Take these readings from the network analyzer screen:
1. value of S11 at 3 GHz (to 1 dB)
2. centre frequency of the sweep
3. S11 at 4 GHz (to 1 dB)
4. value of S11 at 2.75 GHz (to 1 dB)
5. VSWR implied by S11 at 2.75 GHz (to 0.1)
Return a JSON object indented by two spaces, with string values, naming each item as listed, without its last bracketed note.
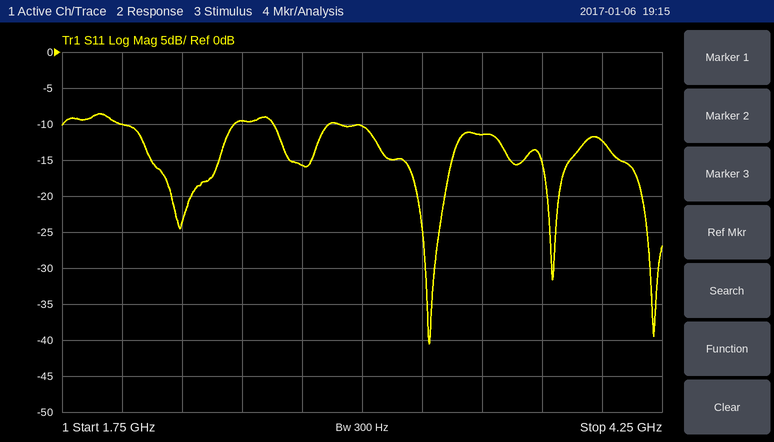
{
  "value of S11 at 3 GHz": "-10 dB",
  "centre frequency of the sweep": "3 GHz",
  "S11 at 4 GHz": "-12 dB",
  "value of S11 at 2.75 GHz": "-16 dB",
  "VSWR implied by S11 at 2.75 GHz": "1.4"
}
